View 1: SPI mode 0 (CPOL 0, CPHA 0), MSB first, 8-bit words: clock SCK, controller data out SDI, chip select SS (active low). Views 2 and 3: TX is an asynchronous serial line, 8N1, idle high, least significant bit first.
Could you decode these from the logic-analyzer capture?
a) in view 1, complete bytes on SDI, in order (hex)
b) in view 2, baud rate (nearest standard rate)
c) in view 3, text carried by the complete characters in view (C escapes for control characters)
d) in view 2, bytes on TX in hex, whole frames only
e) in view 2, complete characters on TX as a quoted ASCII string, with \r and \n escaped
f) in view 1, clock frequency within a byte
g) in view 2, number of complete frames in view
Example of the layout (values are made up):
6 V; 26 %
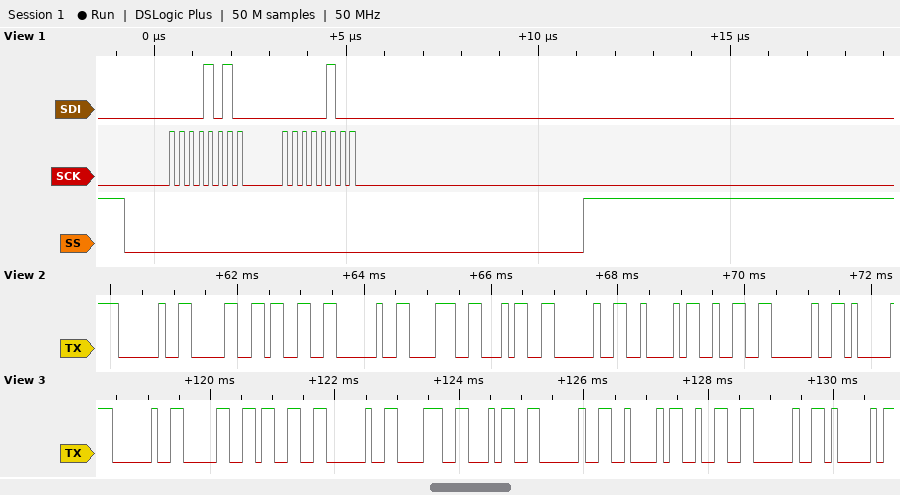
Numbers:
0A 04; 9600 baud; " 03 84 B2 A"; 0x20 0x30 0x33 0x20 0x38 0x34 0x20 0x42 0x32 0x20; " 03 84 B2 "; 4 MHz; 10
